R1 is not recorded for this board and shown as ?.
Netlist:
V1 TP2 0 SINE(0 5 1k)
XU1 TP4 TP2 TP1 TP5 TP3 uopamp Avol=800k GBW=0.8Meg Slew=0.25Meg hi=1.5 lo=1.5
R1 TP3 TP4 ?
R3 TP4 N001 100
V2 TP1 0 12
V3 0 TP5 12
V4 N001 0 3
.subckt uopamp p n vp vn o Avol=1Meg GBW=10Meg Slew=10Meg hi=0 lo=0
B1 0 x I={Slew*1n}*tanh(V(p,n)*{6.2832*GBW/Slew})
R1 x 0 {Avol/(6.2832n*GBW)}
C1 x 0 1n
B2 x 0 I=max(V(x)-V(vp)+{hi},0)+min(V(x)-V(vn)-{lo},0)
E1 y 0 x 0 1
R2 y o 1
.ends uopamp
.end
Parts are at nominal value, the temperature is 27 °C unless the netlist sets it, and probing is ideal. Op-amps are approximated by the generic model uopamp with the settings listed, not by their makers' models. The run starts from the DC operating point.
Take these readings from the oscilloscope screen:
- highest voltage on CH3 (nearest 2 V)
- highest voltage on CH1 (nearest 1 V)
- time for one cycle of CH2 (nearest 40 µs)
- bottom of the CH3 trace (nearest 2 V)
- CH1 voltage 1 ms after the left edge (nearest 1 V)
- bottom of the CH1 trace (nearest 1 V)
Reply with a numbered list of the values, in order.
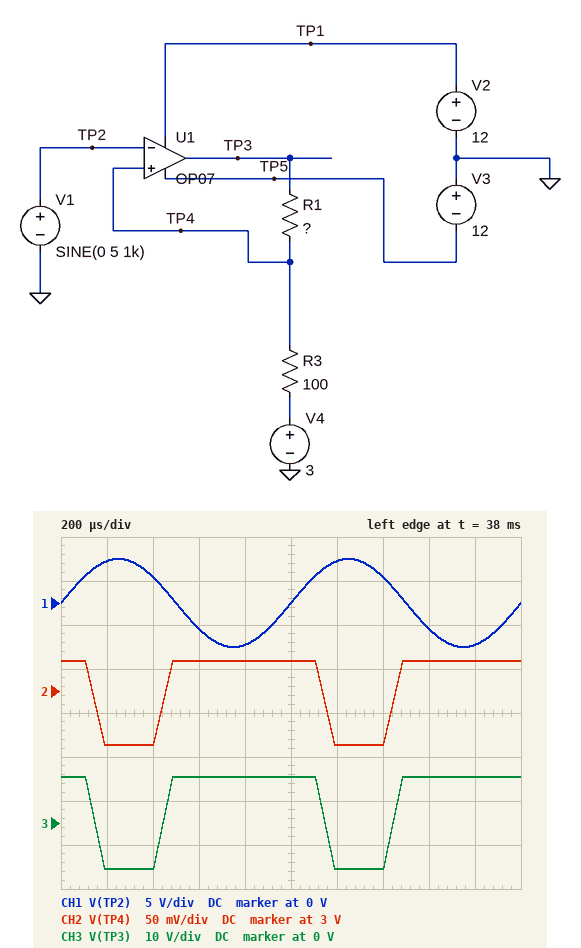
1. 10 V
2. 5 V
3. 1.00 ms
4. -10 V
5. 0 V
6. -5 V
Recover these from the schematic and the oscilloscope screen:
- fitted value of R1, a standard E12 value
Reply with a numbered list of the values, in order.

1. 22 kΩ
